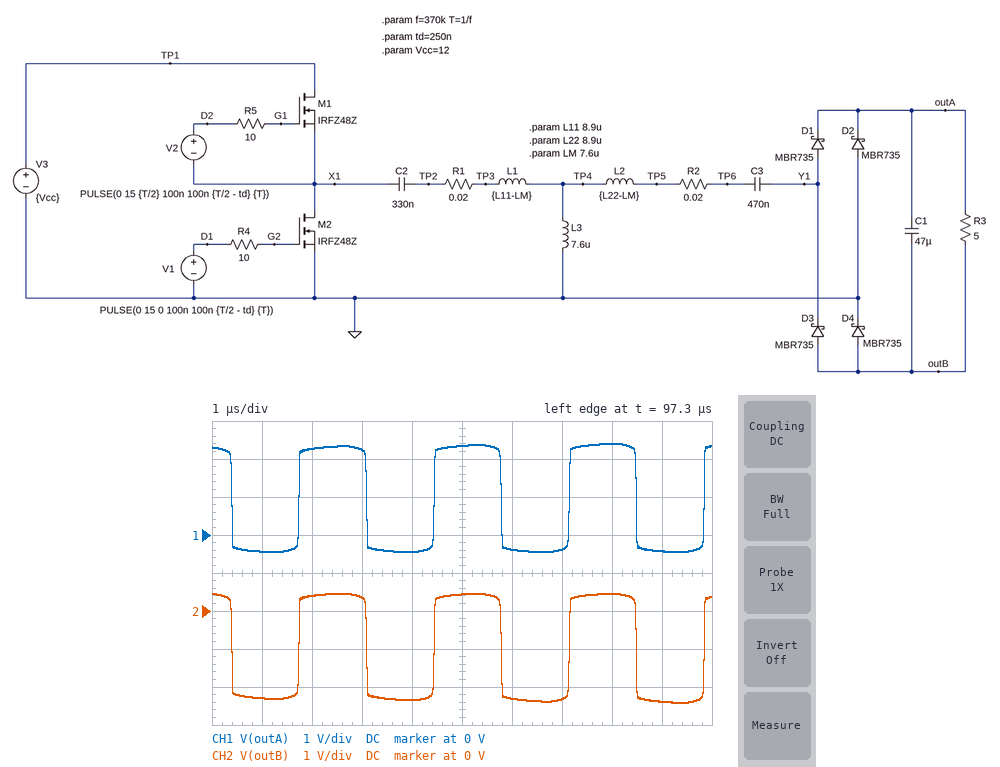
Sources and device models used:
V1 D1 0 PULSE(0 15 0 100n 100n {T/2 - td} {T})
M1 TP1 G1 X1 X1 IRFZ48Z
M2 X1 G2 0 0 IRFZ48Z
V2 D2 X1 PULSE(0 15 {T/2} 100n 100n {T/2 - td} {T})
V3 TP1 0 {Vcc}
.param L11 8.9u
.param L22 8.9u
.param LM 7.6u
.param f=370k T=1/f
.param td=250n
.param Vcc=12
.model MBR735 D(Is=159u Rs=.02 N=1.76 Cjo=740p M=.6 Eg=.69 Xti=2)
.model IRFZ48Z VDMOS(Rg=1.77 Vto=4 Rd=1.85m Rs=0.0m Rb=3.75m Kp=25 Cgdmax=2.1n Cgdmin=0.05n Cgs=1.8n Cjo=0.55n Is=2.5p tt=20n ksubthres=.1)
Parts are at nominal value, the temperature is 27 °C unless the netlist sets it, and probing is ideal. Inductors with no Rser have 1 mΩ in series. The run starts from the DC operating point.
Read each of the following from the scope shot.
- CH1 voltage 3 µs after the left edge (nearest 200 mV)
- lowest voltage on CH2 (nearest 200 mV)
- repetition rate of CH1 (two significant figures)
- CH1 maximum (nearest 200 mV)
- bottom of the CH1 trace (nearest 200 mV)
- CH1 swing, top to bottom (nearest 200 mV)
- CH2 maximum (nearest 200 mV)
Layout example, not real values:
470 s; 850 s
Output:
2.2 V; -2.4 V; 370 kHz; 2.4 V; -400 mV; 2.8 V; 400 mV
